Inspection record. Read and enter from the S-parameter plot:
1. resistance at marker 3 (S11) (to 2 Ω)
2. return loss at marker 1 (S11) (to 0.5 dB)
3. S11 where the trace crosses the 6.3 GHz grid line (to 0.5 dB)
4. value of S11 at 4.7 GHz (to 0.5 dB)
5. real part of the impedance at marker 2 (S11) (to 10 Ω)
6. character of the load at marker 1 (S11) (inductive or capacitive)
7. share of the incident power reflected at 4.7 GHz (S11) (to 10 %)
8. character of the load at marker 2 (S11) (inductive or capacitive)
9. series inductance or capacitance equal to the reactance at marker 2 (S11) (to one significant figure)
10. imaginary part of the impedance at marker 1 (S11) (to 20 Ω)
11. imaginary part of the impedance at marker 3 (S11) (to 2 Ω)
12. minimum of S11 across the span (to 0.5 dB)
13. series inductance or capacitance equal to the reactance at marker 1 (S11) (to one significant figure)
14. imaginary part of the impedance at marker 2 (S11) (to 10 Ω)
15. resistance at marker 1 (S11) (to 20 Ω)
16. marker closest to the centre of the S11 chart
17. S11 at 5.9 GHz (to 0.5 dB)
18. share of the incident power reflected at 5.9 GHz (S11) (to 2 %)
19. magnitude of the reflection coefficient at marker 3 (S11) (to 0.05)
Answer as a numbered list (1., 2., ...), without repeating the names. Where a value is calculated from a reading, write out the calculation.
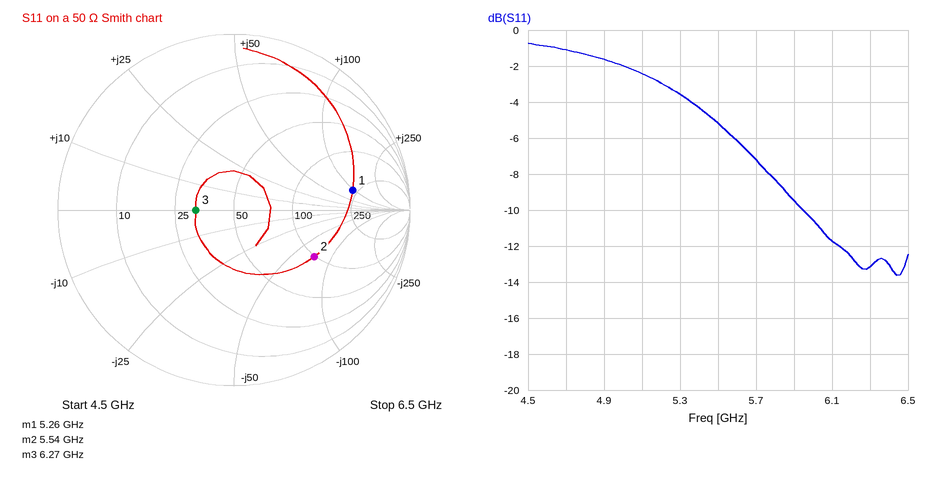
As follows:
1. 32 Ω
2. 3.5 dB
3. -13.0 dB
4. -1.0 dB
5. 100 Ω
6. inductive
7. 10^(-1/10) ≈ 79.4 %, so 80 % to the nearest 10 %
8. capacitive
9. C = 1/(2π × 5.54 GHz × 70 Ω) ≈ 410 fF, so 400 fF to one significant figure
10. +100 Ω
11. 0 Ω
12. -13.5 dB
13. L = 100 Ω/(2π × 5.26 GHz) ≈ 3 nH
14. -70 Ω
15. 220 Ω
16. marker 3
17. -9.5 dB
18. 10^(-9.5/10) ≈ 11.2 %, so 12 % to the nearest 2 %
19. 0.20
